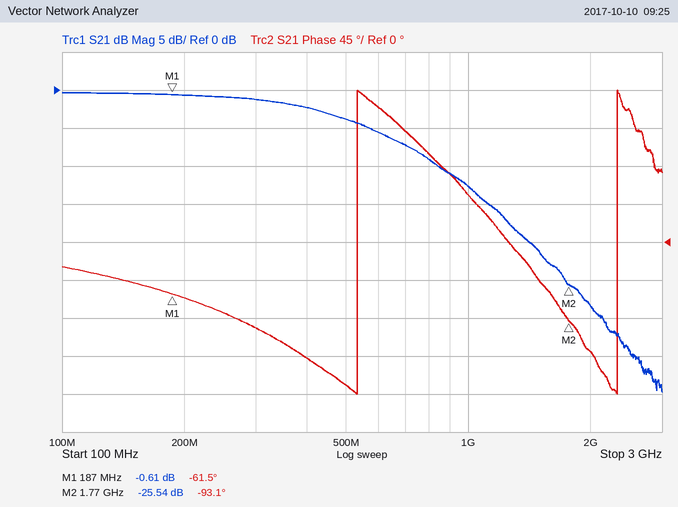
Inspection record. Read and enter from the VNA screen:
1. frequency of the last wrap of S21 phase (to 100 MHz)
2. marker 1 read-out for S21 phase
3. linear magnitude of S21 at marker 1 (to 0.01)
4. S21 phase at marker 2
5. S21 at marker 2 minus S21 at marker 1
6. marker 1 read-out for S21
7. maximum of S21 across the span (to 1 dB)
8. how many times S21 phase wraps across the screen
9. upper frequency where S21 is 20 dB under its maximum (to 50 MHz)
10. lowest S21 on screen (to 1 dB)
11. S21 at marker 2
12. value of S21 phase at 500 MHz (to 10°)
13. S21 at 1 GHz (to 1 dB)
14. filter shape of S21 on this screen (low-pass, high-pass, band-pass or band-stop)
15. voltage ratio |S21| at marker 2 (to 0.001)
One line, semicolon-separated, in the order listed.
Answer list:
2.3 GHz; -61.5°; 0.93; -93.1°; -24.93 dB; -0.61 dB; 0 dB; 2; 1.45 GHz; -40 dB; -25.54 dB; -170°; -13 dB; low-pass; 0.053
